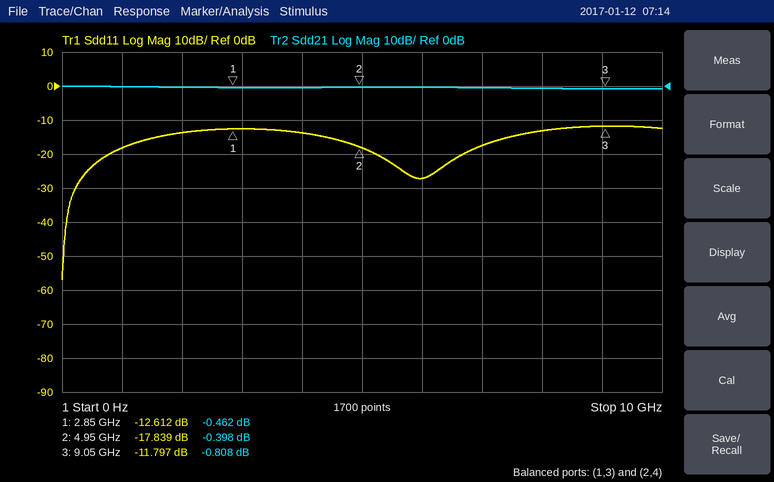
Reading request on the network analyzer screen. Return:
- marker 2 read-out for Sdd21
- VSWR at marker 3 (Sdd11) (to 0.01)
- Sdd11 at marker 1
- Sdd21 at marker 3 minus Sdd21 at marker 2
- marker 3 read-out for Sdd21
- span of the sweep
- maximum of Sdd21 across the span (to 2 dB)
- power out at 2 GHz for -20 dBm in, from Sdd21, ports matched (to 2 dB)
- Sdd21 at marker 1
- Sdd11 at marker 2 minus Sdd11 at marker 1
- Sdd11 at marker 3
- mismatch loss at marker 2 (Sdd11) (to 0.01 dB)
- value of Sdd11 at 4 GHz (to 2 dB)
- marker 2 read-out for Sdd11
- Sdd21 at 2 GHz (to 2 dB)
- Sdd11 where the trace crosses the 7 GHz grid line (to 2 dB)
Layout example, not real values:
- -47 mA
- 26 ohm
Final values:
- -0.398 dB
- 1.69
- -12.612 dB
- -0.410 dB
- -0.808 dB
- 10 GHz
- 0 dB
- -20 dBm
- -0.462 dB
- -5.227 dB
- -11.797 dB
- 0.07 dB
- -14 dB
- -17.839 dB
- 0 dB
- -18 dB
